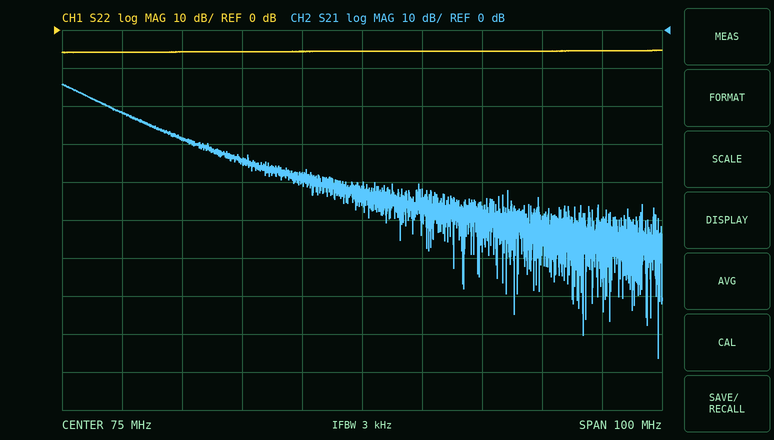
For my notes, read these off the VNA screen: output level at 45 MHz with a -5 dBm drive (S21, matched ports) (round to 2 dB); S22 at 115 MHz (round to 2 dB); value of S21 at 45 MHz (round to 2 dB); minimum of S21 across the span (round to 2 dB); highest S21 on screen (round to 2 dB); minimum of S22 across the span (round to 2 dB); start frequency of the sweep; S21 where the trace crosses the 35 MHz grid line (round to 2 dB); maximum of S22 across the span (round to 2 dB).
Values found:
-34 dBm
-6 dB
-28 dB
-86 dB
-14 dB
-6 dB
25 MHz
-22 dB
-6 dB
